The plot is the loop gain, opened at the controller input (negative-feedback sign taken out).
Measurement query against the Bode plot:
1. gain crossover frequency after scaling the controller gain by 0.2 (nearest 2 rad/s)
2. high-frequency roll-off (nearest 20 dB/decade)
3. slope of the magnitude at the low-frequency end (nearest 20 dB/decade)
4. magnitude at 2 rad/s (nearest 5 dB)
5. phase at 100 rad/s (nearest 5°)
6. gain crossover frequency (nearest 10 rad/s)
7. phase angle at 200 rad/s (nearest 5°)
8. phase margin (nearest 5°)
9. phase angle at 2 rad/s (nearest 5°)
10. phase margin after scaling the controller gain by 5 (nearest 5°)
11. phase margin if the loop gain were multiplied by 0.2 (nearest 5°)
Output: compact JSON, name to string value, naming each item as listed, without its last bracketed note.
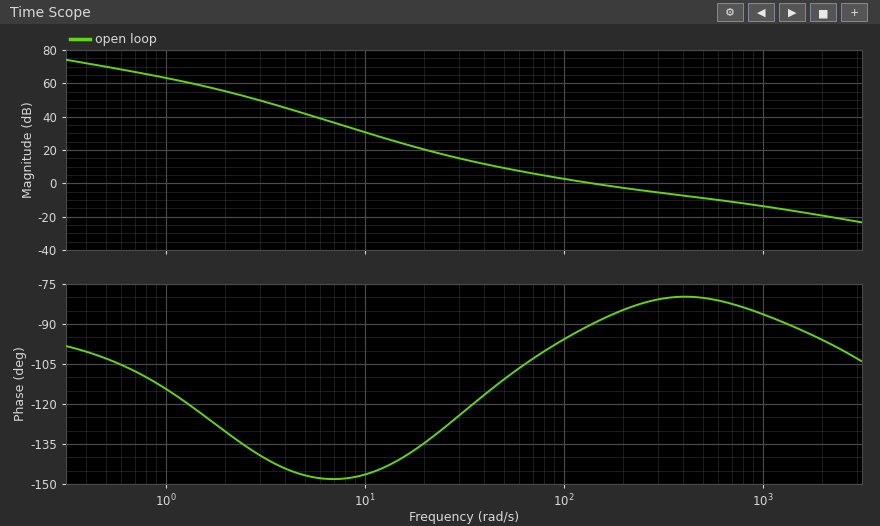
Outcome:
{"gain crossover frequency after scaling the controller gain by 0.2": "32 rad/s", "high-frequency roll-off": "-20 dB/decade", "slope of the magnitude at the low-frequency end": "-20 dB/decade", "magnitude at 2 rad/s": "55 dB", "phase at 100 rad/s": "-95°", "gain crossover frequency": "140 rad/s", "phase angle at 200 rad/s": "-85°", "phase margin": "90°", "phase angle at 2 rad/s": "-130°", "phase margin after scaling the controller gain by 5": "95°", "phase margin if the loop gain were multiplied by 0.2": "60°"}
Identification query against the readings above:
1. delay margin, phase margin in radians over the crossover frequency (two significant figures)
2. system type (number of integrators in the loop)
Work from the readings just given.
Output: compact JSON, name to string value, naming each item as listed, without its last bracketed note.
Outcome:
{"delay margin, phase margin in radians over the crossover frequency": "0.011 s", "system type": "1"}
